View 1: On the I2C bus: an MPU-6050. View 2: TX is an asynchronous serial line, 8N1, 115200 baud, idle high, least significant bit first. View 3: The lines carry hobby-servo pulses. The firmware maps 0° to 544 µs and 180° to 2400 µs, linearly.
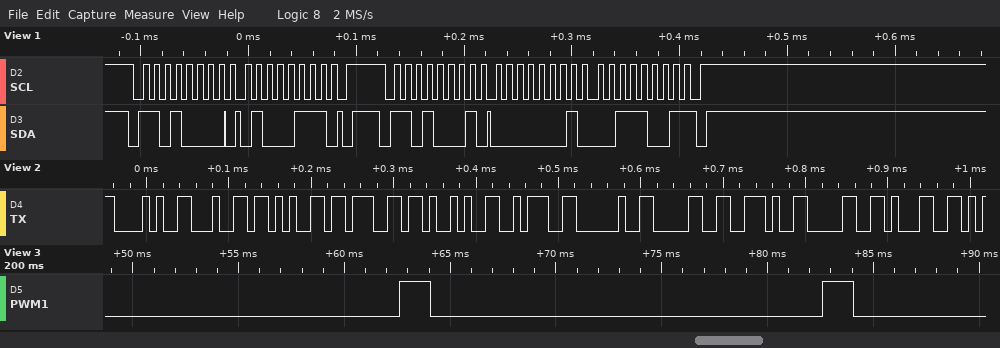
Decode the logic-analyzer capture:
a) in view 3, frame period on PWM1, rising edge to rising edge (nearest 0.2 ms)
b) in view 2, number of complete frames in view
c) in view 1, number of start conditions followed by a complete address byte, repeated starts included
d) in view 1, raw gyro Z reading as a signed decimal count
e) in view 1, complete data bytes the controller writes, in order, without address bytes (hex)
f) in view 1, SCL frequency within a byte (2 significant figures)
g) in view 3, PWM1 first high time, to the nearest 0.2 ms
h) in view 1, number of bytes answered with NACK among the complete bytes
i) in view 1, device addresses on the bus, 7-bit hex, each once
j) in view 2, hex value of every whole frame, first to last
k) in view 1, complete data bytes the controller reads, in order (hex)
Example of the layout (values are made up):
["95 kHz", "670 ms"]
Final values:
["20.0 ms", "11", "2", "313", "47", "100 kHz", "1.4 ms", "1", "0x68", "0x28 0x64 0x65 0x67 0x29 0x3A 0x20 0x30 0x2E 0x30 0x31", "01 39"]
